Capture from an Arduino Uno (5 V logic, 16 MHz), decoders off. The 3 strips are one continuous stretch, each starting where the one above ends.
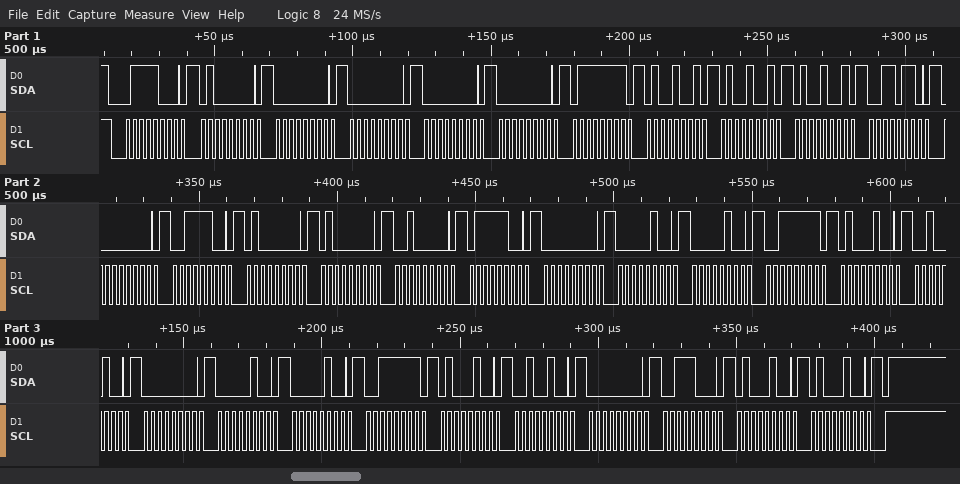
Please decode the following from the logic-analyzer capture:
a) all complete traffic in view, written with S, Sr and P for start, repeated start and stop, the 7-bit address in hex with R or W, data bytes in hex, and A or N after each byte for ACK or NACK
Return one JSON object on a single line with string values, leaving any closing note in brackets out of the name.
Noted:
{"all complete traffic in view, written with S, Sr and P for start, repeated start and stop, the 7-bit address in hex with R or W, data bytes in hex, and A or N after each byte for ACK or NACK": "S 3CW A 40 A 00 A 00 A 00 A 00 A 7F A 49 A 49 A 49 A 36 A 00 A 3C A 40 A 40 A 20 A 7C A 00 A 04 A 04 A 3F A 44 A 24 A 00 A 04 A 04 A 3F A 44 A 24 A 00 A 38 A 44 A 44 A P"}
